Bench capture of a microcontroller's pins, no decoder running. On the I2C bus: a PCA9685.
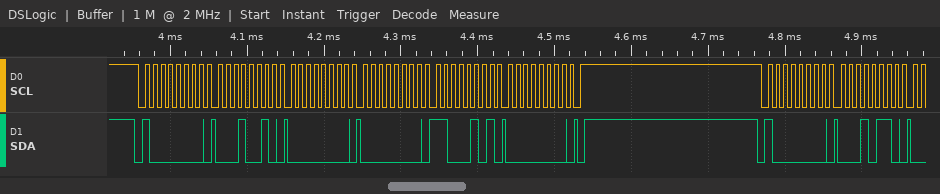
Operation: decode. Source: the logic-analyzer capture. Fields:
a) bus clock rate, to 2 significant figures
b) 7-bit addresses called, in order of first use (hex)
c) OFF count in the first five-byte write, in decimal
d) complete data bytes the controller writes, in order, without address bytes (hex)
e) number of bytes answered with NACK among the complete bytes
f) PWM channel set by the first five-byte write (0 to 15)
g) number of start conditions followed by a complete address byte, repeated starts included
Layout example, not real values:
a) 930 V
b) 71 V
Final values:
a) 100 kHz
b) 0x40
c) 197
d) 12 00 00 C5 00 16
e) 0
f) 3
g) 2
